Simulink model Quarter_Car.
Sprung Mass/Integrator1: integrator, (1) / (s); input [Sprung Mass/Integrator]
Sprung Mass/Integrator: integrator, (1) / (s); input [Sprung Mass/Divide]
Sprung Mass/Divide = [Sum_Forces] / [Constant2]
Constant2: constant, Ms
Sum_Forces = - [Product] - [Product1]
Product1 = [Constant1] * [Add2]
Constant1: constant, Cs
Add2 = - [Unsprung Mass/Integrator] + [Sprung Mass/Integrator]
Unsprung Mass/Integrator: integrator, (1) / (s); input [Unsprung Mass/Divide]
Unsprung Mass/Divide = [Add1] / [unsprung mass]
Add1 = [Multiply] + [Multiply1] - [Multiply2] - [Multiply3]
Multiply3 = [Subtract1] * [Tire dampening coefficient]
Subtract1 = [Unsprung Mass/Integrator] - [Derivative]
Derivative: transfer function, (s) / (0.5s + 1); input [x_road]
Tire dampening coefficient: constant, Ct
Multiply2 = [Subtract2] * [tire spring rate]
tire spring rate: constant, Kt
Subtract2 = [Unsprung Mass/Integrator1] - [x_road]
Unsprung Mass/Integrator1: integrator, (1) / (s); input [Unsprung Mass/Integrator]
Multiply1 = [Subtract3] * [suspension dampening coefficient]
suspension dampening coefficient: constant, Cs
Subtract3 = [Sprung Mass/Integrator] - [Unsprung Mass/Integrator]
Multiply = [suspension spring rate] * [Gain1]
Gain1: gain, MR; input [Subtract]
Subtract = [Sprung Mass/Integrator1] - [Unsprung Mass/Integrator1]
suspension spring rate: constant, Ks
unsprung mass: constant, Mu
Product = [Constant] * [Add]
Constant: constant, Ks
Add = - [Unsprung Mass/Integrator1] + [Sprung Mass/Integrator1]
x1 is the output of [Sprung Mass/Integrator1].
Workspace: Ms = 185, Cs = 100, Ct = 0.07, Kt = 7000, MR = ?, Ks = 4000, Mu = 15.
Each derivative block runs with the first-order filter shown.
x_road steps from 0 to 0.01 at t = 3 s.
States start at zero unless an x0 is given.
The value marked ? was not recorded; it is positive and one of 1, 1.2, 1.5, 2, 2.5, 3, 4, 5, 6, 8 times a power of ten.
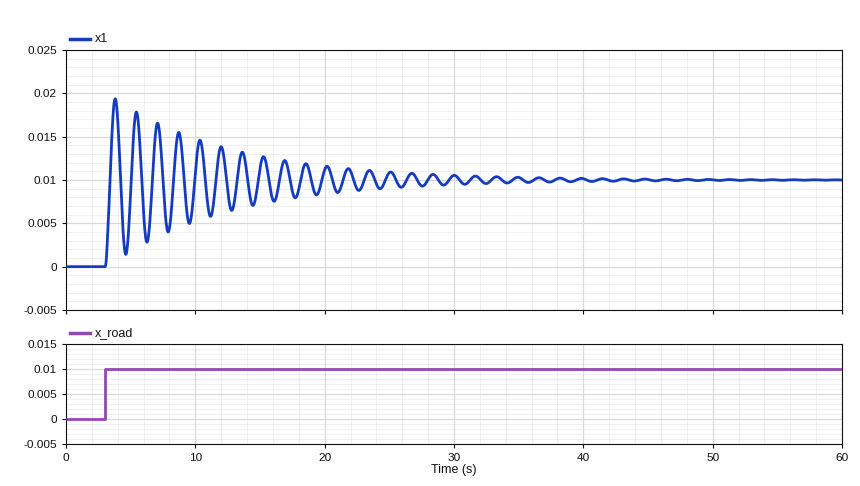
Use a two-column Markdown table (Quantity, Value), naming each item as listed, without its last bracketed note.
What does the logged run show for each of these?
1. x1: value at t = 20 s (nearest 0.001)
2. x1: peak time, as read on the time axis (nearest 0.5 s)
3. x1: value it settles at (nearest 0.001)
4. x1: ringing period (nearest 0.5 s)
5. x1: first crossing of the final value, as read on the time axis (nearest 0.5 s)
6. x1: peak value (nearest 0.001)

| Quantity | Value |
|---|---|
| x1: value at t = 20 s | 0.011 |
| x1: peak time, as read on the time axis | 4.0 s |
| x1: value it settles at | 0.010 |
| x1: ringing period | 1.5 s |
| x1: first crossing of the final value, as read on the time axis | 3.5 s |
| x1: peak value | 0.019 |
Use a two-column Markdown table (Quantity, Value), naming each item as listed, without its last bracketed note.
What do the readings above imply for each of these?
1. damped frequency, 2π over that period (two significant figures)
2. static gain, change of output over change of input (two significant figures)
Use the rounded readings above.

| Quantity | Value |
|---|---|
| damped frequency, 2π over that period | 4.2 rad/s |
| static gain, change of output over change of input | 1.0 |
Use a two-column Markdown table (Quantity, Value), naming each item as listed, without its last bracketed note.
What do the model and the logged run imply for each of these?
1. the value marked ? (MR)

| Quantity | Value |
|---|---|
| the value marked ? | 0.8 |
